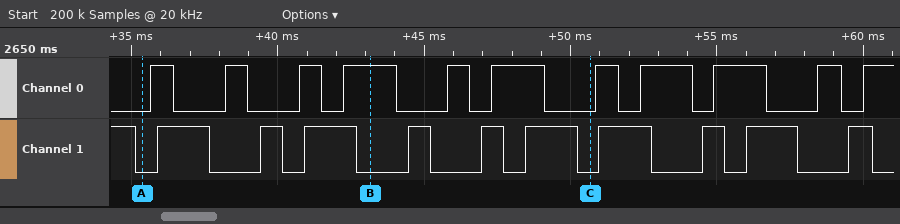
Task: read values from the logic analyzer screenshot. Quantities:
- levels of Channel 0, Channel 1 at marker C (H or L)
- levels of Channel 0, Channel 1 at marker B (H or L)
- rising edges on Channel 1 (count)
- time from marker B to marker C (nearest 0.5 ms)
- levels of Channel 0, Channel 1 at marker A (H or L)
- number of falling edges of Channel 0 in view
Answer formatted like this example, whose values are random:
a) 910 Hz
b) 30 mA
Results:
a) Channel 0=L, Channel 1=L
b) Channel 0=H, Channel 1=L
c) 10
d) 7.5 ms
e) Channel 0=L, Channel 1=L
f) 10
